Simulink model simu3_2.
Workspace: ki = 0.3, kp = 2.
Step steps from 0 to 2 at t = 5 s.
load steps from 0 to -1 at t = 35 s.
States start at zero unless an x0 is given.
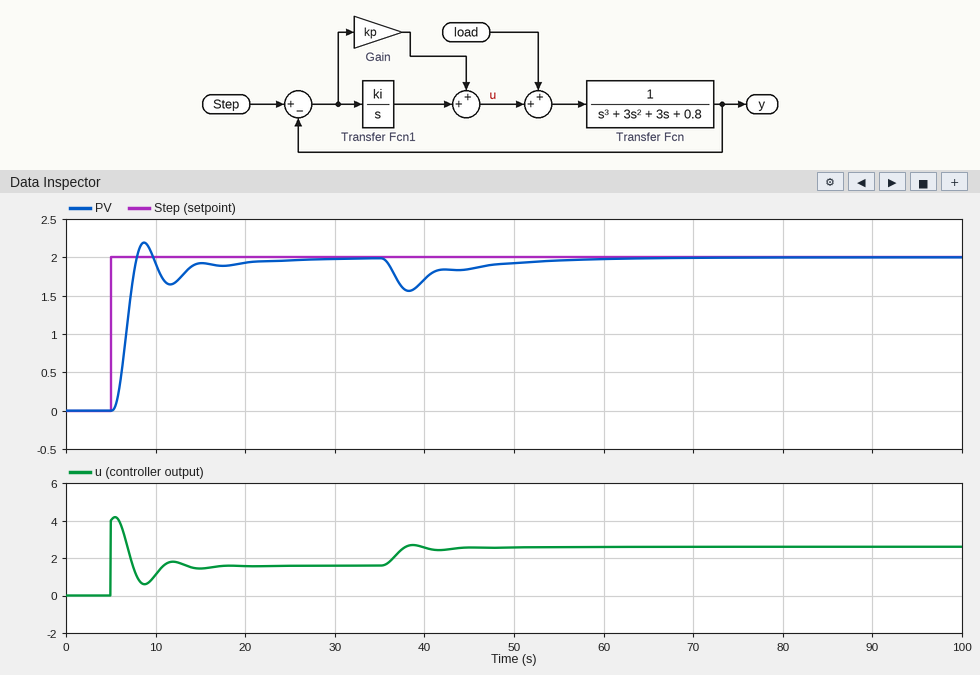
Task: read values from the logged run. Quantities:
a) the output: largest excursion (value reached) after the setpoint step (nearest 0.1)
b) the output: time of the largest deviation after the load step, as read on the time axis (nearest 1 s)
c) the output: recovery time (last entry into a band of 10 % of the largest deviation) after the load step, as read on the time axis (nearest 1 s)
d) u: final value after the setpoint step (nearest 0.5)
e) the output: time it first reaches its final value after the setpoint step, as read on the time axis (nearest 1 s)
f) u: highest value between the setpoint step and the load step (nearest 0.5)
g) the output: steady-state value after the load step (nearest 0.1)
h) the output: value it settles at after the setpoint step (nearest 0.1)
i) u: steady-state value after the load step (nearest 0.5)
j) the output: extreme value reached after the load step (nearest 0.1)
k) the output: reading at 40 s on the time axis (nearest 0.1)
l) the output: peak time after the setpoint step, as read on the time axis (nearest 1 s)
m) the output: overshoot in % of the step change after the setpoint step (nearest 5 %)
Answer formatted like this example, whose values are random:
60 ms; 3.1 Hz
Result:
2.2; 38 s; 55 s; 1.5; 8 s; 4.0; 2.0; 2.0; 2.5; 1.6; 1.7; 9 s; 10 %
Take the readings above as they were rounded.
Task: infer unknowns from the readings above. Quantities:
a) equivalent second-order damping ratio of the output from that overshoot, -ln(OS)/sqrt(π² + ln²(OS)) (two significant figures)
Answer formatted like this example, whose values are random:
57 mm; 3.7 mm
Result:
0.59
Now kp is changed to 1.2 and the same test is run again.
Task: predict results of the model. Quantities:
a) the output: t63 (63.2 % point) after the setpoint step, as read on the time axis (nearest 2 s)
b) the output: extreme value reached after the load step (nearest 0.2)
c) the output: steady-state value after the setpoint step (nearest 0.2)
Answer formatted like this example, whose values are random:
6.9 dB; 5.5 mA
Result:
8 s; 1.4; 2.0
